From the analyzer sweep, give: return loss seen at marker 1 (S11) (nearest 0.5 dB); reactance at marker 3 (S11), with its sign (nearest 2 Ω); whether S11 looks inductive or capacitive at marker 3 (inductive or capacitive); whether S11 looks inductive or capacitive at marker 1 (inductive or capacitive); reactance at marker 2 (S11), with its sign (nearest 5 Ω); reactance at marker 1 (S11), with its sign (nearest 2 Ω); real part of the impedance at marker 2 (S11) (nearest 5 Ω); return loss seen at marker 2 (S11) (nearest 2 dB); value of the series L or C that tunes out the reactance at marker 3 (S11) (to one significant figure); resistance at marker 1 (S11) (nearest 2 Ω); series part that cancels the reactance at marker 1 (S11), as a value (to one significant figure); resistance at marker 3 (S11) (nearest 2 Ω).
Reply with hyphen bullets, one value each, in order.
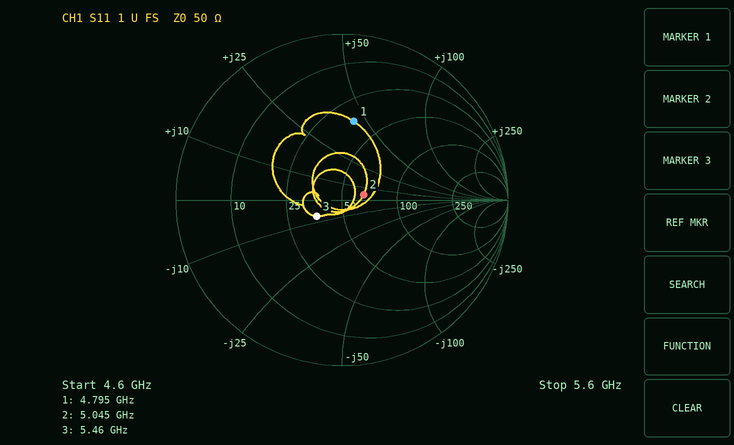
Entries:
- 6.5 dB
- -8 Ω
- capacitive
- inductive
- +5 Ω
- +44 Ω
- 65 Ω
- 18 dB
- 200 pH
- 36 Ω
- 800 fF
- 36 Ω
